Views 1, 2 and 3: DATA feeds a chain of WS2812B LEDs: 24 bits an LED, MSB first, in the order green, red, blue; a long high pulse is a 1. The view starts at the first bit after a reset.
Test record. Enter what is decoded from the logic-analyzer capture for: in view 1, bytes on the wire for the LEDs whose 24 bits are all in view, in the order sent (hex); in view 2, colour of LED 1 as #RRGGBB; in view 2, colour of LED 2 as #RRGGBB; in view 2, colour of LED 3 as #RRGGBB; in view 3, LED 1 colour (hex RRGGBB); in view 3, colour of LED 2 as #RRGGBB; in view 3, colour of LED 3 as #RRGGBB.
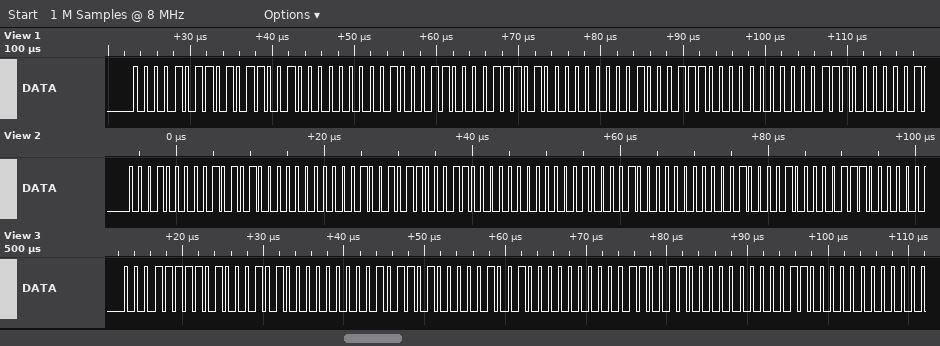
0B 59 00 46 1D 00 47 00 1C
#541000
#184B00
#004221
#451F00
#095A00
#003330
